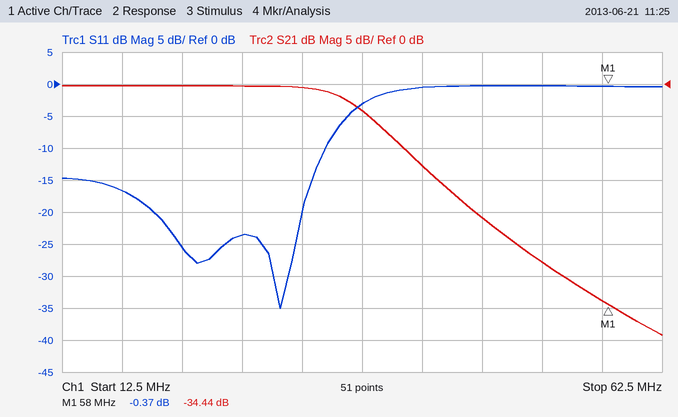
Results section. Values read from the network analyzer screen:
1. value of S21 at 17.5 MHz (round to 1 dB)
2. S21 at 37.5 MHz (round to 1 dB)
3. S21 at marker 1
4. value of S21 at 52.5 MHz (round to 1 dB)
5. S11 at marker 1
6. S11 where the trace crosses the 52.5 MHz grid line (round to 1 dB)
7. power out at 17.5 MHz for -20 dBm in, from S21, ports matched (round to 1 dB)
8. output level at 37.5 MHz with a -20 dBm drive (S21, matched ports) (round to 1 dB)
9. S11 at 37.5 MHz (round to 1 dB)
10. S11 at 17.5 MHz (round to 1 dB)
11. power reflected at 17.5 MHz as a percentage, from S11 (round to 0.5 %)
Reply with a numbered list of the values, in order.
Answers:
1. 0 dB
2. -4 dB
3. -34.44 dB
4. -28 dB
5. -0.37 dB
6. 0 dB
7. -20 dBm
8. -24 dBm
9. -3 dB
10. -17 dB
11. 2.0 %
